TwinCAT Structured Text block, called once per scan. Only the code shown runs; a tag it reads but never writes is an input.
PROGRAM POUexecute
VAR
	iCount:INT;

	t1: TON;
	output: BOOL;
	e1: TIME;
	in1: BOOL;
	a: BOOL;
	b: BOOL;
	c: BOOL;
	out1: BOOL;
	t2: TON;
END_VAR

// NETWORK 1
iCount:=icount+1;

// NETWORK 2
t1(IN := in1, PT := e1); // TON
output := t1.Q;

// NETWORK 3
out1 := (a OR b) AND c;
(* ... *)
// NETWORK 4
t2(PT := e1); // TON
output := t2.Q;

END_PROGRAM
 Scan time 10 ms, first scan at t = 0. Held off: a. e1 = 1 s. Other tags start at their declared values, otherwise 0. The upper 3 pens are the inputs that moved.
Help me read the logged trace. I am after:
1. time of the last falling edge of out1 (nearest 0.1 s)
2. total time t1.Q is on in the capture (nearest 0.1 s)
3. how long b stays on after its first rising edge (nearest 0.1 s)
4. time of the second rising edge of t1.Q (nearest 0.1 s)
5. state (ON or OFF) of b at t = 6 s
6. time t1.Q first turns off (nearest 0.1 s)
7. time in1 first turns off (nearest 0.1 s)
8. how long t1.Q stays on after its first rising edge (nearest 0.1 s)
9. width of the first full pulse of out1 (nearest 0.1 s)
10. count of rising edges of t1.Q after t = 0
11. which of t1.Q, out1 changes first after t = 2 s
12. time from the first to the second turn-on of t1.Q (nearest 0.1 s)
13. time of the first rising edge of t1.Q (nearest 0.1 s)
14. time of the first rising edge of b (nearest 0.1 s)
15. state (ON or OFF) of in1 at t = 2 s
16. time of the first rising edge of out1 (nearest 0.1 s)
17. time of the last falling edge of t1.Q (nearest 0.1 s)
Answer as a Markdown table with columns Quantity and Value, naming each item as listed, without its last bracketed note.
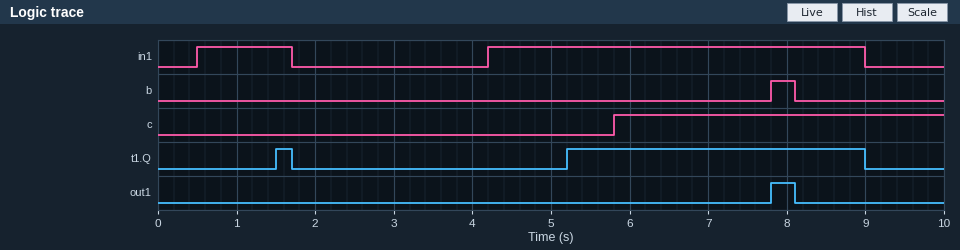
| Quantity | Value |
|---|---|
| time of the last falling edge of out1 | 8.1 s |
| total time t1.Q is on in the capture | 4.0 s |
| how long b stays on after its first rising edge | 0.3 s |
| time of the second rising edge of t1.Q | 5.2 s |
| state (ON or OFF) of b at t = 6 s | OFF |
| time t1.Q first turns off | 1.7 s |
| time in1 first turns off | 1.7 s |
| how long t1.Q stays on after its first rising edge | 0.2 s |
| width of the first full pulse of out1 | 0.3 s |
| count of rising edges of t1.Q after t = 0 | 2 |
| which of t1.Q, out1 changes first after t = 2 s | t1.Q |
| time from the first to the second turn-on of t1.Q | 3.7 s |
| time of the first rising edge of t1.Q | 1.5 s |
| time of the first rising edge of b | 7.8 s |
| state (ON or OFF) of in1 at t = 2 s | OFF |
| time of the first rising edge of out1 | 7.8 s |
| time of the last falling edge of t1.Q | 9.0 s |
